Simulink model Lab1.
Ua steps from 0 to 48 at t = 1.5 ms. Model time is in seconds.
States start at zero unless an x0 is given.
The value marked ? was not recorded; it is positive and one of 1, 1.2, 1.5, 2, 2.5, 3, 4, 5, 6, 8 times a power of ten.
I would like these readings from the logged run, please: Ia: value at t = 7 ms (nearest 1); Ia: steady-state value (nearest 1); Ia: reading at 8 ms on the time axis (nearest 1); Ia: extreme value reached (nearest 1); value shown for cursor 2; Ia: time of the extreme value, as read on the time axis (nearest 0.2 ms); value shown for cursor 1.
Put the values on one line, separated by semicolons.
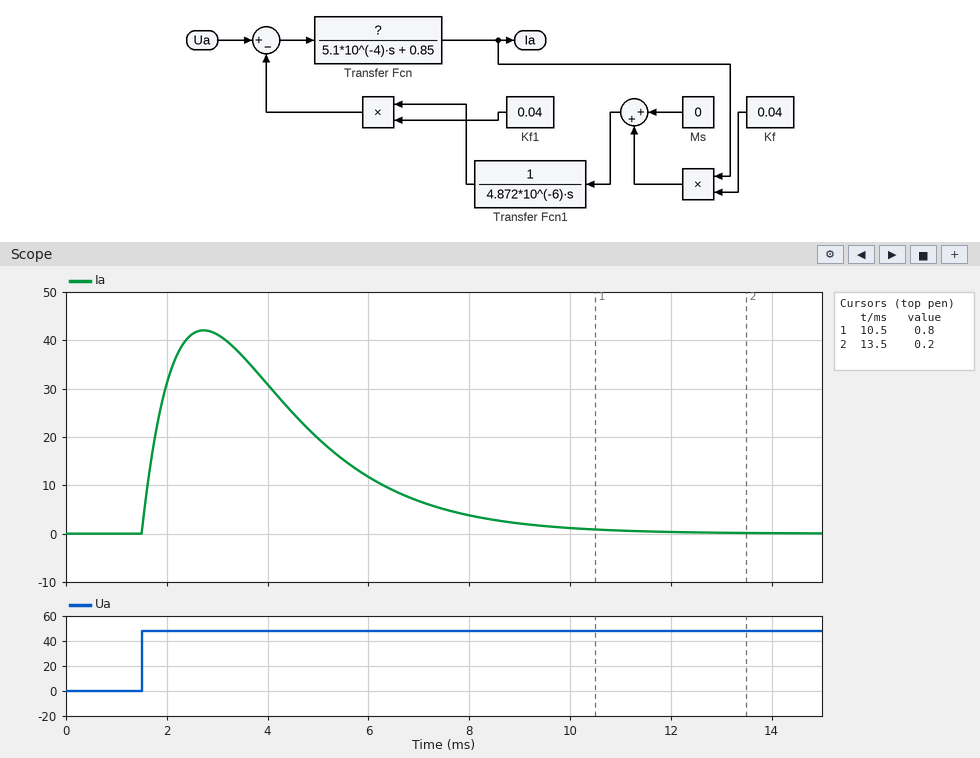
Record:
7; 0; 4; 42; 0.2; 2.8 ms; 0.8
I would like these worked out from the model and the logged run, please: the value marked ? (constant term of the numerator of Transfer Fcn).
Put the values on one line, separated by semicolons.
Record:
1
